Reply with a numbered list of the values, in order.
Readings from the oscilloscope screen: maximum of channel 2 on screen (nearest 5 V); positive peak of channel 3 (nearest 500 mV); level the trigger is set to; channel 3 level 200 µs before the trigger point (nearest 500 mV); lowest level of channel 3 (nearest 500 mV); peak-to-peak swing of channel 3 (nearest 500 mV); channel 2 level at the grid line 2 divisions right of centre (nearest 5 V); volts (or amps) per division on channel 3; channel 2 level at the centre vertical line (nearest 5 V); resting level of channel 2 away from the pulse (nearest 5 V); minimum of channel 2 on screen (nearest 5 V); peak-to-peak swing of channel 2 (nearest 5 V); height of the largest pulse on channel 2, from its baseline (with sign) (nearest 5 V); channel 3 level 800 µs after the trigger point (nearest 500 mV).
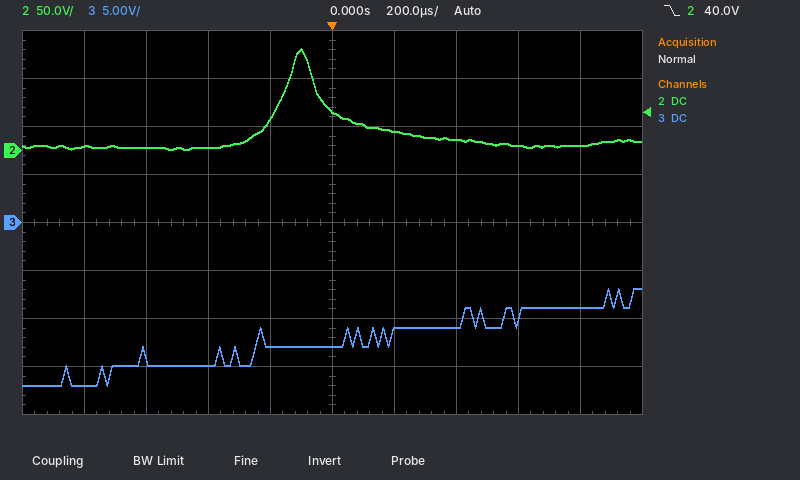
1. 105 V
2. -7.0 V
3. 40.0 V
4. -13.0 V
5. -17.0 V
6. 10.0 V
7. 10 V
8. 5 V
9. 40 V
10. 5 V
11. 0 V
12. 105 V
13. +100 V
14. -9.0 V
